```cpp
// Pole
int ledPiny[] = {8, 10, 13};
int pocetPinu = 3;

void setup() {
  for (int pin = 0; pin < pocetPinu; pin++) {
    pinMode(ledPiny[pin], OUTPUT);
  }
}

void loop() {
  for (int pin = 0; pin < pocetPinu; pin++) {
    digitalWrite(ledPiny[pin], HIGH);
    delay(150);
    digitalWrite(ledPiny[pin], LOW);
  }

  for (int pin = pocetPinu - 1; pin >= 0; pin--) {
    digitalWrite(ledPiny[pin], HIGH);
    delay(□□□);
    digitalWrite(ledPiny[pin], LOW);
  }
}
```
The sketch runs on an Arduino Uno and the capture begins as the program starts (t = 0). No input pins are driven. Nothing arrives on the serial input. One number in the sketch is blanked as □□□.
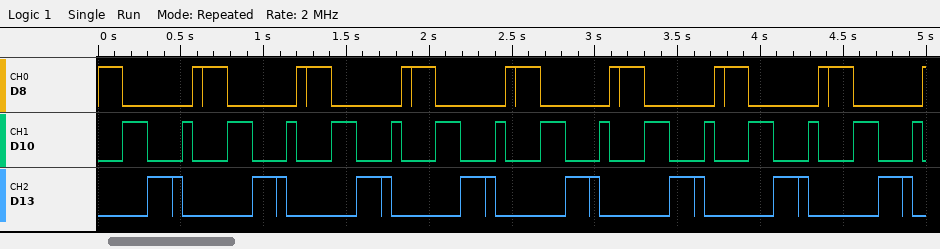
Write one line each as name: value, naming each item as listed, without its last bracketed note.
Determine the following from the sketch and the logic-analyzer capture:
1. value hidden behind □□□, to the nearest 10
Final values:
value hidden behind □□□, to the nearest 10: 60
